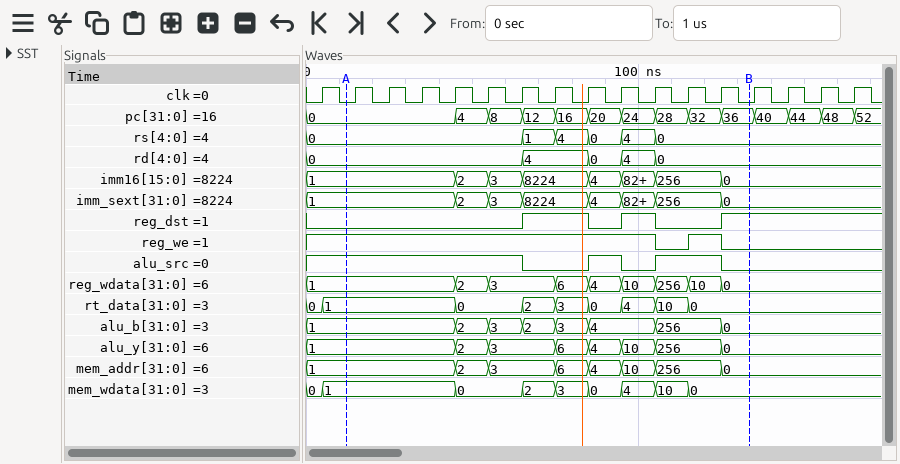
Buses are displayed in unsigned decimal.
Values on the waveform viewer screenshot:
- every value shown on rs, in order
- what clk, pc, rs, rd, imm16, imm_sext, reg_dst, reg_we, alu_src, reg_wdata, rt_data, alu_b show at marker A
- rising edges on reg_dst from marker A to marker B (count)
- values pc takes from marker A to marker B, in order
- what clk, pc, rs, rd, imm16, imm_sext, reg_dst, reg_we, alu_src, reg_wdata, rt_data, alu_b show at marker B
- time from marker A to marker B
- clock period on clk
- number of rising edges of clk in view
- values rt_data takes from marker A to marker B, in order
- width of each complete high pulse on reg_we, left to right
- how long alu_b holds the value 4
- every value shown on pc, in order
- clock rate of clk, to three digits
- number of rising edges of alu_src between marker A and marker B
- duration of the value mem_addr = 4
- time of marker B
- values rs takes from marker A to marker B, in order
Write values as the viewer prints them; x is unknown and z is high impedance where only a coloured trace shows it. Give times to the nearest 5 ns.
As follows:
0, 1, 4, 0, 4, 0
clk=0, pc=0, rs=0, rd=0, imm16=1, imm_sext=1, reg_dst=0, reg_we=1, alu_src=1, reg_wdata=1, rt_data=1, alu_b=1
3
0, 4, 8, 12, 16, 20, 24, 28, 32, 36
clk=0, pc=36, rs=0, rd=0, imm16=0, imm_sext=0, reg_dst=1, reg_we=0, alu_src=0, reg_wdata=0, rt_data=0, alu_b=0
120 ns
10 ns
17
1, 0, 2, 3, 0, 4, 10, 0
10 ns
20 ns
0, 4, 8, 12, 16, 20, 24, 28, 32, 36, 40, 44, 48, 52
100 MHz
2
10 ns
135 ns
0, 1, 4, 0, 4, 0
